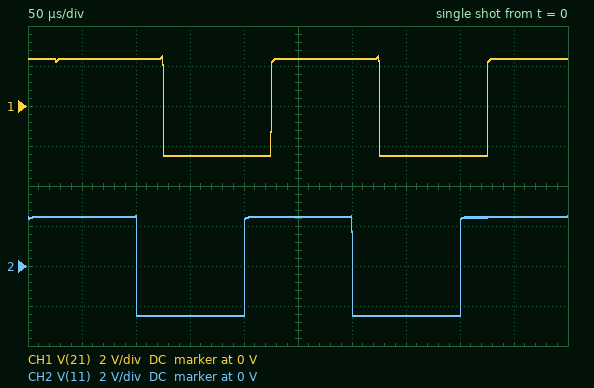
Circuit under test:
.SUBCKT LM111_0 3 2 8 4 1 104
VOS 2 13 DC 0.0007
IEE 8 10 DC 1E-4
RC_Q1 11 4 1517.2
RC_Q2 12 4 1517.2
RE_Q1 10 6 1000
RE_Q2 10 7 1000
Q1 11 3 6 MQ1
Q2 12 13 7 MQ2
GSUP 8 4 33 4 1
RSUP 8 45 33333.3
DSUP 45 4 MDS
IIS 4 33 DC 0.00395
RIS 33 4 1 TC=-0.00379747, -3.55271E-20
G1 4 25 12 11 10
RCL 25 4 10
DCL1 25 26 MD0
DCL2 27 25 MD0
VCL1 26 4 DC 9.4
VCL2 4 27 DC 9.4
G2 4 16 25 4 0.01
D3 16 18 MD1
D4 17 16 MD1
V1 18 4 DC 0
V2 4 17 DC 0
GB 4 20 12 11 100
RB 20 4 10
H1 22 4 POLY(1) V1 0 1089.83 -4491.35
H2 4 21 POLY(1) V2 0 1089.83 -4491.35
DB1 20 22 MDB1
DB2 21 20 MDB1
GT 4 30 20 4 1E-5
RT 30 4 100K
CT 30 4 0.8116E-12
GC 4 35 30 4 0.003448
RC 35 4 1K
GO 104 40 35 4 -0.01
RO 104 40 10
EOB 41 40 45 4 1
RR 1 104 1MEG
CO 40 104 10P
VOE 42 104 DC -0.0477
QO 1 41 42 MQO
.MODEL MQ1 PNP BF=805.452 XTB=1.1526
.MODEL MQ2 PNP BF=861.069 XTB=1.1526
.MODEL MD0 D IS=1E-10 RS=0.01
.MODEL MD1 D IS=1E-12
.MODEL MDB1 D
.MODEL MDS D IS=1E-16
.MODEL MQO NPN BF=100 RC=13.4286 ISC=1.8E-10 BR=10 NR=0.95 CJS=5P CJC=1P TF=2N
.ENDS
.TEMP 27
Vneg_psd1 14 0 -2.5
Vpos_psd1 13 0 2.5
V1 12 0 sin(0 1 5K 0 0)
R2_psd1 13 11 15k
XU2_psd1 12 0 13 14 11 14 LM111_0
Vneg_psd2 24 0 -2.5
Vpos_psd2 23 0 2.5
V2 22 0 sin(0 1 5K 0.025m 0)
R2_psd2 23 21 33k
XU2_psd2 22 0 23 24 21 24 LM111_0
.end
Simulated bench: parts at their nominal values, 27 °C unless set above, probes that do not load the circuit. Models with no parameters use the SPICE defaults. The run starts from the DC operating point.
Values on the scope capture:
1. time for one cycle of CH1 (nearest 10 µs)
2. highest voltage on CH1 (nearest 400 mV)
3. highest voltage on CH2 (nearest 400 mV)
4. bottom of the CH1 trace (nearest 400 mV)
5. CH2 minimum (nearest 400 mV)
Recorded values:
200 µs
2.4 V
2.4 V
-2.4 V
-2.4 V
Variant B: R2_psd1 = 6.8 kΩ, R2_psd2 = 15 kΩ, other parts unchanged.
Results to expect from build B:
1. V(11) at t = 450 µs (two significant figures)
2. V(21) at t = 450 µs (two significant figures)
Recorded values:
2.5 V
2.4 V
